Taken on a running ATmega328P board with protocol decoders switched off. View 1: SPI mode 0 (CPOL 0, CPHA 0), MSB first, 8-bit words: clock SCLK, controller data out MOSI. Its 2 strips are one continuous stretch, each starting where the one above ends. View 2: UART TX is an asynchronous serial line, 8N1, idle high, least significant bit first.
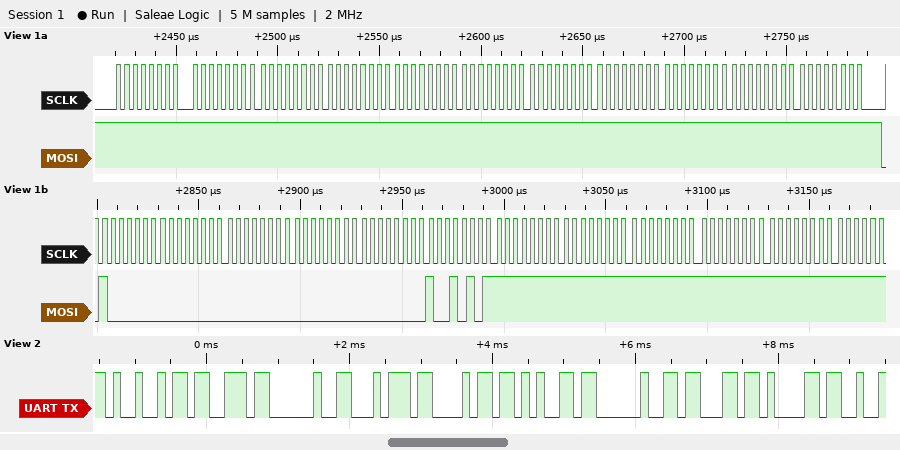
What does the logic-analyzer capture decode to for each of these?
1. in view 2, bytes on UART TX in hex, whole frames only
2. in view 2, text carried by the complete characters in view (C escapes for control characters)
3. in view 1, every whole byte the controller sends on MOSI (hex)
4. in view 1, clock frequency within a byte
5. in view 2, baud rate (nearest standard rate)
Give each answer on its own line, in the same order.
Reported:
49 73 20 74 68 65 20 63 61
"Is the ca"
FF FF FF FF FF FF FF FF FF FF FF 40 00 00 00 00 95 FF FF FF FF FF
250 kHz
9600 baud
